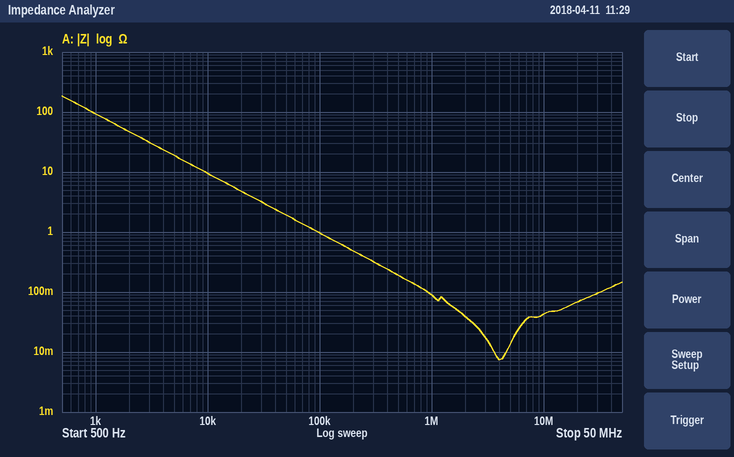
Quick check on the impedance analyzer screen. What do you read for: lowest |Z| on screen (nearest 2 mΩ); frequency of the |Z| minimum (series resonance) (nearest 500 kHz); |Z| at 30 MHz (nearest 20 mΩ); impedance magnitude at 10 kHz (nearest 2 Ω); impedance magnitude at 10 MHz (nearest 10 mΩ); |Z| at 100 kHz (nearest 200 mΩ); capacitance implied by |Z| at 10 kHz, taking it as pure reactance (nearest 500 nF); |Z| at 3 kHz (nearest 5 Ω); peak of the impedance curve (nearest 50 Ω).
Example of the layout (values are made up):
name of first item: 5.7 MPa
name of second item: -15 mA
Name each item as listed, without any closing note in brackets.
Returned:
lowest |Z| on screen: 8 mΩ
frequency of the |Z| minimum (series resonance): 4.0 MHz
|Z| at 30 MHz: 100 mΩ
impedance magnitude at 10 kHz: 10 Ω
impedance magnitude at 10 MHz: 40 mΩ
|Z| at 100 kHz: 1.0 Ω
capacitance implied by |Z| at 10 kHz, taking it as pure reactance: 1.5 µF
|Z| at 3 kHz: 30 Ω
peak of the impedance curve: 200 Ω
